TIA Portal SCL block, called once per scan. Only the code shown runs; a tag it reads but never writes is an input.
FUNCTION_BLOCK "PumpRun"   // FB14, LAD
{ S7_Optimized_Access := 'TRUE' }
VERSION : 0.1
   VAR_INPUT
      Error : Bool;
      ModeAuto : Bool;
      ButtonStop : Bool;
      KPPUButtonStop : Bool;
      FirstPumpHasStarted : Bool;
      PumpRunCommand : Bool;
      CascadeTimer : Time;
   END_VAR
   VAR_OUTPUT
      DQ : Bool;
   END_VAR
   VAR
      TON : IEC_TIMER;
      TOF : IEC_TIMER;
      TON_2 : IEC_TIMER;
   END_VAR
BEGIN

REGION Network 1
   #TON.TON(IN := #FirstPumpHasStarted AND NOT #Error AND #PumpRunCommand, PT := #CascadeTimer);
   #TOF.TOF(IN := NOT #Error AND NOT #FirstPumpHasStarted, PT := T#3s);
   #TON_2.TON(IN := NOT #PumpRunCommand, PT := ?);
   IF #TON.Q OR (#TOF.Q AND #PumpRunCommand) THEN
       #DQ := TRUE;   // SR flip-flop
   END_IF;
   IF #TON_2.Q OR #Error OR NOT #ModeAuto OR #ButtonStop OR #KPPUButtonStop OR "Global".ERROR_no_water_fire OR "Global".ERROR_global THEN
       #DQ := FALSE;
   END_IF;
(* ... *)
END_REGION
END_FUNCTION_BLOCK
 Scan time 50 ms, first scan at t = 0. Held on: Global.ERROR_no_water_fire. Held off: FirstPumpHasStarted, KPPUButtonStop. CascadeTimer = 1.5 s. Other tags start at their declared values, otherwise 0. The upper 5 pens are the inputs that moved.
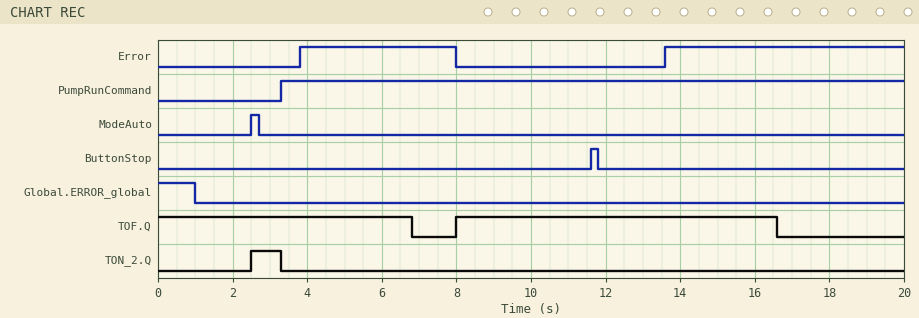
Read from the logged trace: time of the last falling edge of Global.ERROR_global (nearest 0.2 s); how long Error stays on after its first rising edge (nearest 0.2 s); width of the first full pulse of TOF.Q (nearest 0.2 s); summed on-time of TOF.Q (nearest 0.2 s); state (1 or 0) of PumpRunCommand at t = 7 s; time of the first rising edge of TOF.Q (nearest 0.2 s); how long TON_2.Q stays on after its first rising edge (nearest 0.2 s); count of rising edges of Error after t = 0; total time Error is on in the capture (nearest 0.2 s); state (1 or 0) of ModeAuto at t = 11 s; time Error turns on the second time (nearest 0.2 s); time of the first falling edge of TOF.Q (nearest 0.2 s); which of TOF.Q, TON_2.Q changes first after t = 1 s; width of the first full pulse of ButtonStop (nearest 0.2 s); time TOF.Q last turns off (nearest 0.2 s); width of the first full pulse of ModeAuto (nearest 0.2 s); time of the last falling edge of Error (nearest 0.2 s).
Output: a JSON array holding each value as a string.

["1.0 s", "4.2 s", "8.6 s", "15.4 s", "1", "8.0 s", "0.8 s", "2", "10.6 s", "0", "13.6 s", "6.8 s", "TON_2.Q", "0.2 s", "16.6 s", "0.2 s", "8.0 s"]
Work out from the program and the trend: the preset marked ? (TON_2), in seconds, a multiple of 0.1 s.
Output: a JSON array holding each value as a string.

["2.5 s"]
